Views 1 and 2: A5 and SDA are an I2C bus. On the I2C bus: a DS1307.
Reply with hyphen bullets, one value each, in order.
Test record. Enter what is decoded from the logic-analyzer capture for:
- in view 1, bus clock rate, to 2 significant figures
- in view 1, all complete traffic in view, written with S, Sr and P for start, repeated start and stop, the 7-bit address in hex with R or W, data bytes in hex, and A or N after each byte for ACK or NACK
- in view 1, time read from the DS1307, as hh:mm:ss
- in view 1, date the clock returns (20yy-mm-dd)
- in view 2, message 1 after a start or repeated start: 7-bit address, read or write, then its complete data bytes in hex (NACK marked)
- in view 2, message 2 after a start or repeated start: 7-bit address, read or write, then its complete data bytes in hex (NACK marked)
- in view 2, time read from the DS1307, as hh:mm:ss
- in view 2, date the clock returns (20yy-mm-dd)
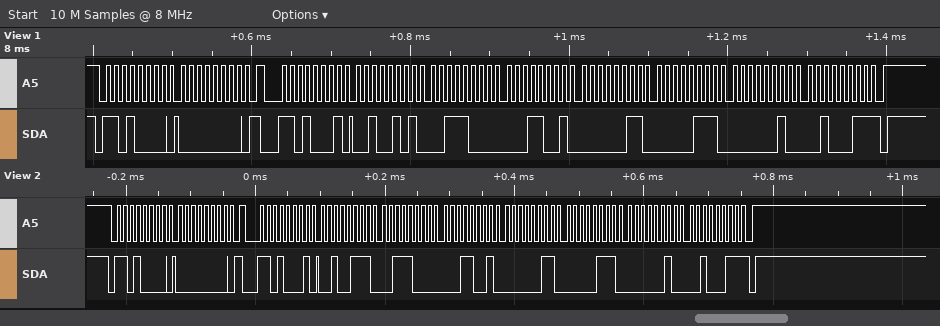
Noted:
- 100 kHz
- S 68W A 00 A Sr 68R A 25 A 38 A 19 A 03 A 07 A 02 A 23 N P
- 19:38:25
- 2023-02-07
- 0x68 write: 00
- 0x68 read: 27 38 19 03 07 02 23 NACK
- 19:38:27
- 2023-02-07
